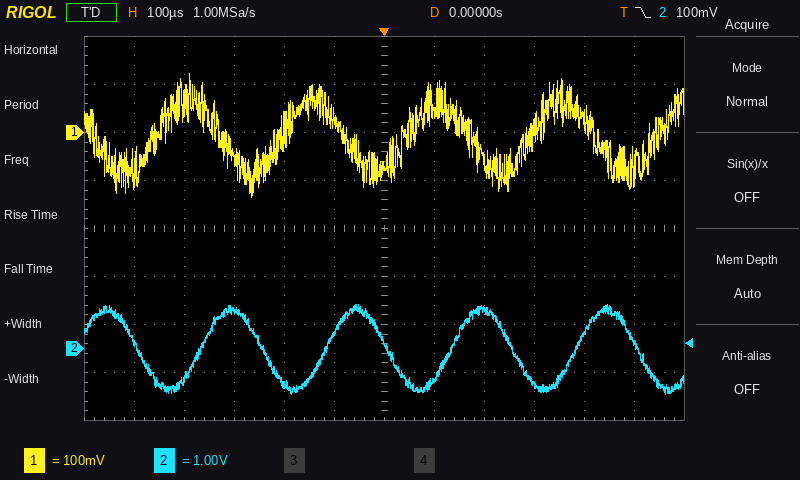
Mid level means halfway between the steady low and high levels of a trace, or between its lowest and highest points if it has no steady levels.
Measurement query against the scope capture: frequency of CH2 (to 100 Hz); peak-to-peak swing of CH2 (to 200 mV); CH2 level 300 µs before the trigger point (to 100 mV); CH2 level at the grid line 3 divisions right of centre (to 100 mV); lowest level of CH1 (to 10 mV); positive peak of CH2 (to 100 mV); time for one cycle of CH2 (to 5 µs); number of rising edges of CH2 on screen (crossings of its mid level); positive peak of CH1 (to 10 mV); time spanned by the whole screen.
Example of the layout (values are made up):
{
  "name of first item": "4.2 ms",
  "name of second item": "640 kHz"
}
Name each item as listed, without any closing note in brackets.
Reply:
{
  "frequency of CH2": "4.0 kHz",
  "peak-to-peak swing of CH2": "1.8 V",
  "CH2 level 300 µs before the trigger point": "800 mV",
  "CH2 level at the grid line 3 divisions right of centre": "-700 mV",
  "lowest level of CH1": "-130 mV",
  "positive peak of CH2": "900 mV",
  "time for one cycle of CH2": "250 µs",
  "number of rising edges of CH2 on screen": "4",
  "positive peak of CH1": "120 mV",
  "time spanned by the whole screen": "1.2 ms"
}
